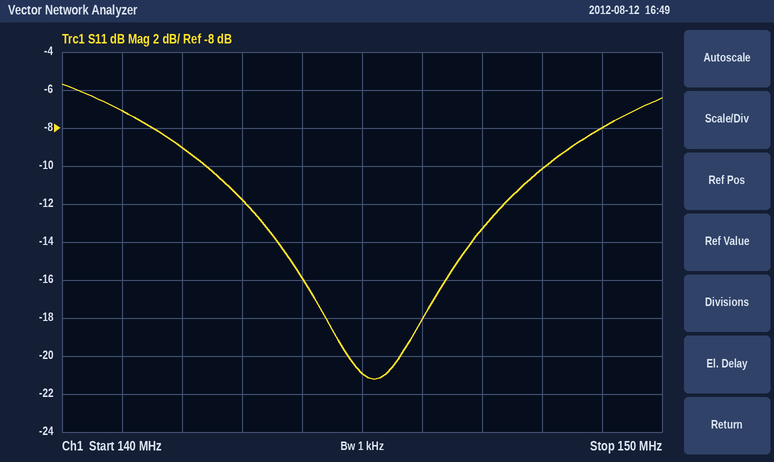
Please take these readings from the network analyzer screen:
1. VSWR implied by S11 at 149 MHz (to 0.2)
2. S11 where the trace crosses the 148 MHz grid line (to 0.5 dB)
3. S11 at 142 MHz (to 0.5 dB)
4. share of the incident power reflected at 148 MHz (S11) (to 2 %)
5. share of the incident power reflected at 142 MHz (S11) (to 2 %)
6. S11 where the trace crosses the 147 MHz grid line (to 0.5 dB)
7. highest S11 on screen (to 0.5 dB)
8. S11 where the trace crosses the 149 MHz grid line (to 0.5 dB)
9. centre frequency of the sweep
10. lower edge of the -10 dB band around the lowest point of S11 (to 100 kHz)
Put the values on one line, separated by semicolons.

2.4; -10.0 dB; -9.0 dB; 10 %; 12 %; -13.5 dB; -5.5 dB; -8.0 dB; 145 MHz; 142.4 MHz
